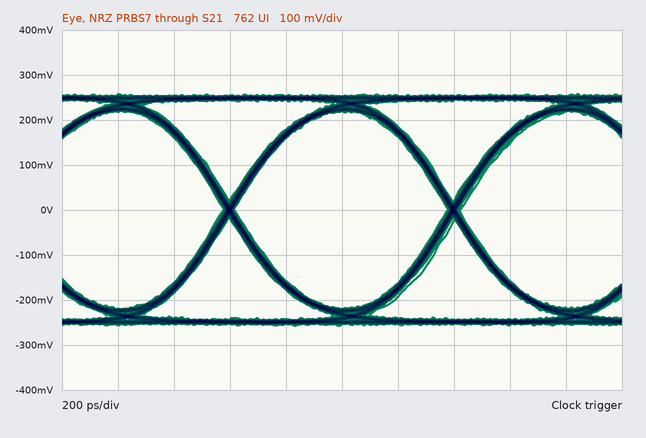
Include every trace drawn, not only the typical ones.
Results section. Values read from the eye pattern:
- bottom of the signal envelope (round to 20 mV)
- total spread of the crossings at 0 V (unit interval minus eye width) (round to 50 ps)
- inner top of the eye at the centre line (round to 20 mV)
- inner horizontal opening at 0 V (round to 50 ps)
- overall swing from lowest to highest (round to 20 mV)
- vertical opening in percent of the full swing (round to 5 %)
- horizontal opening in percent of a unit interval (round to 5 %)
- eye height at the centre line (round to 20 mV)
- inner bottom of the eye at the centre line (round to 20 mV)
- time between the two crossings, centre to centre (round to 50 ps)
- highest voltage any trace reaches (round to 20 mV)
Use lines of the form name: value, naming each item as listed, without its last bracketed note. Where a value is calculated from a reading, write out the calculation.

bottom of the signal envelope: -260 mV
total spread of the crossings at 0 V (unit interval minus eye width): 50 ps
inner top of the eye at the centre line: 220 mV
inner horizontal opening at 0 V: 750 ps
overall swing from lowest to highest: 520 mV
vertical opening in percent of the full swing: 440 mV / 520 mV ≈ 85 %
horizontal opening in percent of a unit interval: 750 ps / 800 ps ≈ 93.7 %, so 95 % to the nearest 5 %
eye height at the centre line: 440 mV
inner bottom of the eye at the centre line: -220 mV
time between the two crossings, centre to centre: 800 ps
highest voltage any trace reaches: 260 mV
